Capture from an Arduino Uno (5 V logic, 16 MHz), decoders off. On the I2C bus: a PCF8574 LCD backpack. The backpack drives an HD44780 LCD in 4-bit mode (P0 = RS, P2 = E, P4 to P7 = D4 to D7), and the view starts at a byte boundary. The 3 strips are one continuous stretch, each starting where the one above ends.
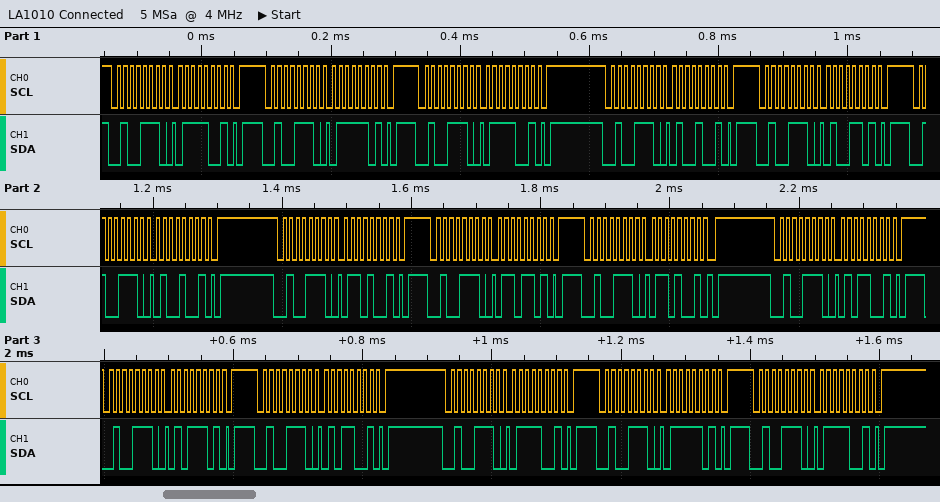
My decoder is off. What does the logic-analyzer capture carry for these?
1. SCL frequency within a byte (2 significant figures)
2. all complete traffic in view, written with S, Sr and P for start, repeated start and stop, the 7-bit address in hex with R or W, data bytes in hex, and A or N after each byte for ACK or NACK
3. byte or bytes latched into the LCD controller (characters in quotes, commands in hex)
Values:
100 kHz
S 27W A 79 A P S 27W A 7D A P S 27W A 79 A P S 27W A 49 A P S 27W A 4D A P S 27W A 49 A P S 27W A 69 A P S 27W A 6D A P S 27W A 69 A P S 27W A 59 A P S 27W A 5D A P S 27W A 59 A P S 27W A 79 A P S 27W A 7D A P S 27W A 79 A P
't' 'e'
